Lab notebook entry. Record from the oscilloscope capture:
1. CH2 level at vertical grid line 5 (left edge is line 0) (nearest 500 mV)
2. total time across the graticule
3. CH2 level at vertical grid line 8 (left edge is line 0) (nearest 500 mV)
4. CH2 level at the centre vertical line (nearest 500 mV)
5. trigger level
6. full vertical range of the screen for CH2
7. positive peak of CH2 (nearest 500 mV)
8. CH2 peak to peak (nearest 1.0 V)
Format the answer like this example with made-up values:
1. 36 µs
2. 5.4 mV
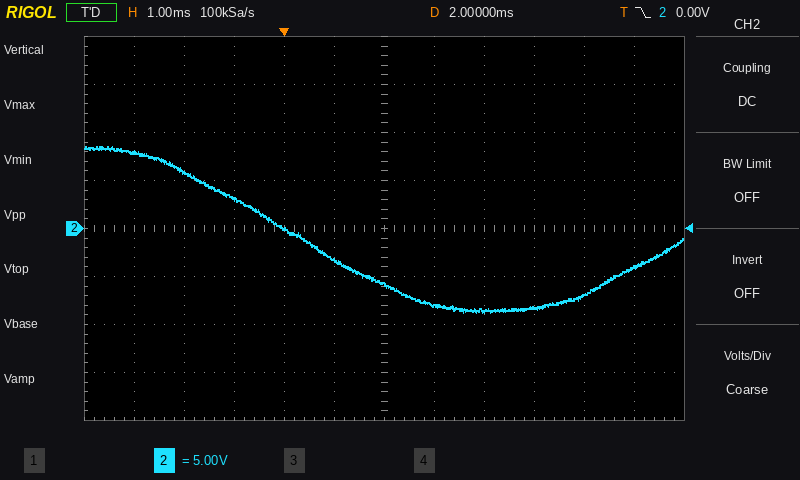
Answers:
1. -3.5 V
2. 12 ms
3. -8.5 V
4. -6.0 V
5. 0.00 V
6. 40 V
7. 8.5 V
8. 17.0 V
